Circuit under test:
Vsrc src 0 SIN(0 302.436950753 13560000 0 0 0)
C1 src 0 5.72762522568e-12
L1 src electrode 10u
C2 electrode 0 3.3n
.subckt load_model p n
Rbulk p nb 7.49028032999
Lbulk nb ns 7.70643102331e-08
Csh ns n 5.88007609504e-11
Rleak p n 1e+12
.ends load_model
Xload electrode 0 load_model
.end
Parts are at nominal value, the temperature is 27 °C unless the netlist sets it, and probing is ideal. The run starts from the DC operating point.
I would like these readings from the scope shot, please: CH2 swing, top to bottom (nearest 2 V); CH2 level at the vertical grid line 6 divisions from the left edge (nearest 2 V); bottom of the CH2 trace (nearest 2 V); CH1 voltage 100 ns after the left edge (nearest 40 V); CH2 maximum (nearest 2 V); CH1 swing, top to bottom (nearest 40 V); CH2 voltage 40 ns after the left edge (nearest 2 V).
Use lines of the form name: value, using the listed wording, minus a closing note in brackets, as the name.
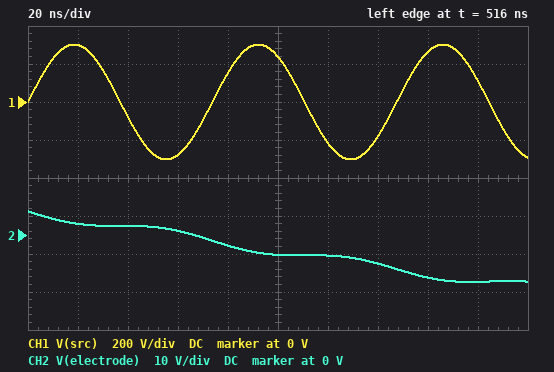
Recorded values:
CH2 swing, top to bottom: 18 V
CH2 level at the vertical grid line 6 divisions from the left edge: -6 V
bottom of the CH2 trace: -12 V
CH1 voltage 100 ns after the left edge: 240 V
CH2 maximum: 6 V
CH1 swing, top to bottom: 600 V
CH2 voltage 40 ns after the left edge: 2 V
